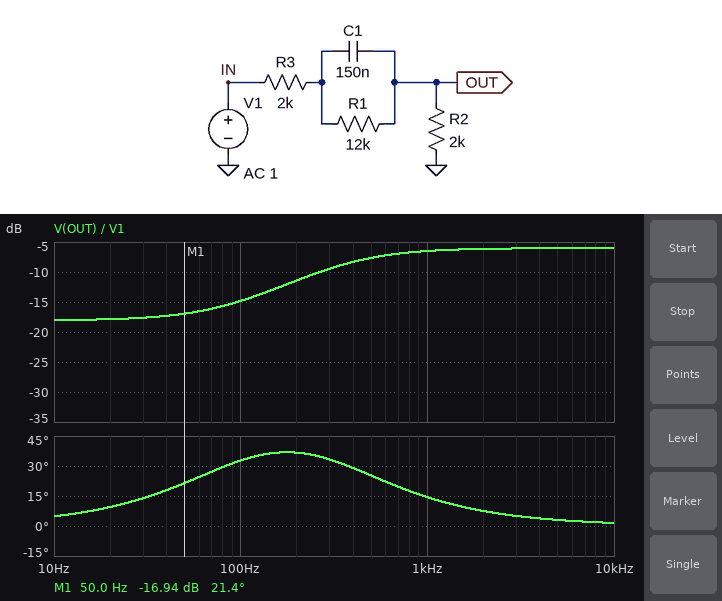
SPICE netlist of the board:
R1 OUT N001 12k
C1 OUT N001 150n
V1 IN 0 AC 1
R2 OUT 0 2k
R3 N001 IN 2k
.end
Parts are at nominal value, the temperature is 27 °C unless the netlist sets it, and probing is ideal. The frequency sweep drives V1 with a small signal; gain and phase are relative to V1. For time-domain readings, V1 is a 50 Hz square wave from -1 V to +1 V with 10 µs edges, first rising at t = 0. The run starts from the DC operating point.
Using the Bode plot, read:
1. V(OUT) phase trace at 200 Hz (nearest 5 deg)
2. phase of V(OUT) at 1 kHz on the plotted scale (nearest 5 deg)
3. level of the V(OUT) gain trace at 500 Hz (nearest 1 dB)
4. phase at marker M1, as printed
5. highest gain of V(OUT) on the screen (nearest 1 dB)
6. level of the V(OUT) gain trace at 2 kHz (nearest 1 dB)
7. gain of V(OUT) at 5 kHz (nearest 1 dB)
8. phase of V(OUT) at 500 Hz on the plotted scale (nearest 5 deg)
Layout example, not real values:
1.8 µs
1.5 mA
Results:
35 deg
15 deg
-8 dB
21.4 deg
-6 dB
-6 dB
-6 dB
25 deg
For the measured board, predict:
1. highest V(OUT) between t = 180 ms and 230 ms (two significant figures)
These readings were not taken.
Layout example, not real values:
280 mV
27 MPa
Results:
870 mV
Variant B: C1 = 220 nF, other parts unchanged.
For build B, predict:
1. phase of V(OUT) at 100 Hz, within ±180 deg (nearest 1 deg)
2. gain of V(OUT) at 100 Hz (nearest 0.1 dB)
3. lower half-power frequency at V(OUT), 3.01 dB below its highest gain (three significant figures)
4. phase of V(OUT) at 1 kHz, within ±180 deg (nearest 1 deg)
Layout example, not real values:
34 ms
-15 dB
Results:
36 deg
-13.0 dB
226 Hz
10 deg
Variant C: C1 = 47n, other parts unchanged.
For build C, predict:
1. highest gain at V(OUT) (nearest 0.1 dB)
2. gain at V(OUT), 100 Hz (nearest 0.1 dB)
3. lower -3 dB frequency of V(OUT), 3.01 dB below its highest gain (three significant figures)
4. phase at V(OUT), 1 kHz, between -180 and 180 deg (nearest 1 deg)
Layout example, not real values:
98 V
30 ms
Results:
-6.0 dB
-17.6 dB
1.06 kHz
33 deg
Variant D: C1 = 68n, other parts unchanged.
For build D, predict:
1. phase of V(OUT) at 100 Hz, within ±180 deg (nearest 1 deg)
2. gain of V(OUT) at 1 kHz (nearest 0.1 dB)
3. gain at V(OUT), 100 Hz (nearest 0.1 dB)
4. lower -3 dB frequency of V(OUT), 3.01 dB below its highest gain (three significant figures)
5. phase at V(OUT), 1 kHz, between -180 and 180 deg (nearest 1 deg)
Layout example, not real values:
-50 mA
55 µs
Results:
20 deg
-7.9 dB
-17.1 dB
730 Hz
27 deg
